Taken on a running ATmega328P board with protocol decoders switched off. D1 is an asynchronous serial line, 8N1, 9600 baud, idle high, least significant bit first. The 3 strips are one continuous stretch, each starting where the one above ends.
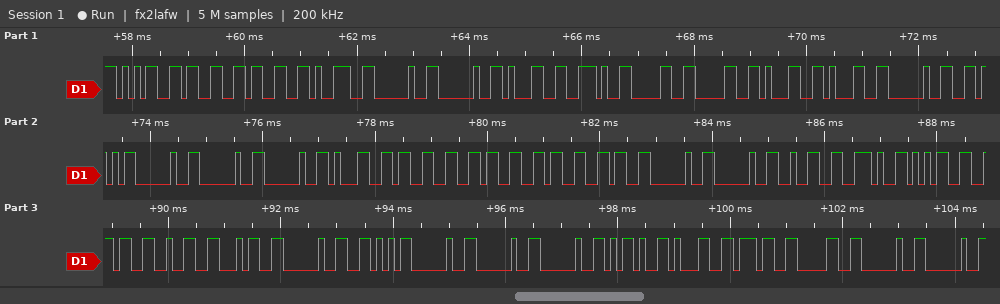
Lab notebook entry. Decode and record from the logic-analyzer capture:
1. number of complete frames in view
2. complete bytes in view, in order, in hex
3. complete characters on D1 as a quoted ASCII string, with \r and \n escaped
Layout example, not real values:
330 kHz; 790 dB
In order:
41; 35 33 33 39 20 20 31 2E 30 30 31 31 20 56 20 20 20 31 33 36 36 36 20 20 32 2E 35 36 32 34 20 56 20 20 20 2D 31 37 30 20 20; "5339  1.0011 V   13666  2.5624 V   -170  "
